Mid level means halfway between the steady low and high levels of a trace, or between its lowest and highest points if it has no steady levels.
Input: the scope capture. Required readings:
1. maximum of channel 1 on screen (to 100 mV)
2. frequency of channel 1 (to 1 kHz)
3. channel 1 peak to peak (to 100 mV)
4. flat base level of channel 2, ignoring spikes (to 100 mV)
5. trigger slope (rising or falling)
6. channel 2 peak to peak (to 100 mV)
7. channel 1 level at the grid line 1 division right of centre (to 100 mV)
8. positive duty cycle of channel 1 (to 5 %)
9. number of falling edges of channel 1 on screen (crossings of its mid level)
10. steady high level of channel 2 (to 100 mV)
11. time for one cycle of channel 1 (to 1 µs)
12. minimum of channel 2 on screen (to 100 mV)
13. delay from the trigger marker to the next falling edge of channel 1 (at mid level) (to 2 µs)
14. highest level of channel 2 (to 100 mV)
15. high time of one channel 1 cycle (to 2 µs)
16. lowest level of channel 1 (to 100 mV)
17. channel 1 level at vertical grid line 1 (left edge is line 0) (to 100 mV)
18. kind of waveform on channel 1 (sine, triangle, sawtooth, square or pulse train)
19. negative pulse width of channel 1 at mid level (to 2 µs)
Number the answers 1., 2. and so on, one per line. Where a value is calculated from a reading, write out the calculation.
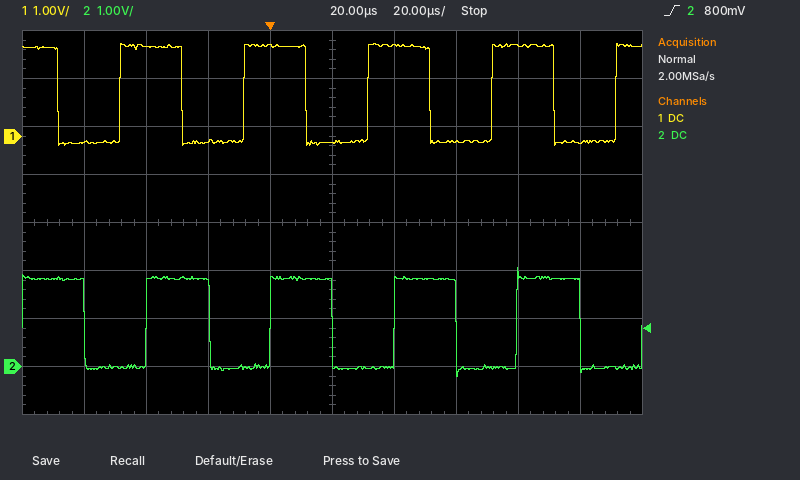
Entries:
1. 1.9 V
2. 1 / 40 µs ≈ 25 kHz
3. 1.9 V − (-200 mV) = 2.1 V
4. 0.0 V
5. rising
6. 2.1 V − (-200 mV) = 2.3 V
7. 1.9 V
8. 20 µs / 40 µs ≈ 50 %
9. 5
10. 1.8 V
11. 40 µs
12. -200 mV
13. 12 µs
14. 2.1 V
15. 20 µs
16. -200 mV
17. -100 mV
18. square
19. 20 µs
